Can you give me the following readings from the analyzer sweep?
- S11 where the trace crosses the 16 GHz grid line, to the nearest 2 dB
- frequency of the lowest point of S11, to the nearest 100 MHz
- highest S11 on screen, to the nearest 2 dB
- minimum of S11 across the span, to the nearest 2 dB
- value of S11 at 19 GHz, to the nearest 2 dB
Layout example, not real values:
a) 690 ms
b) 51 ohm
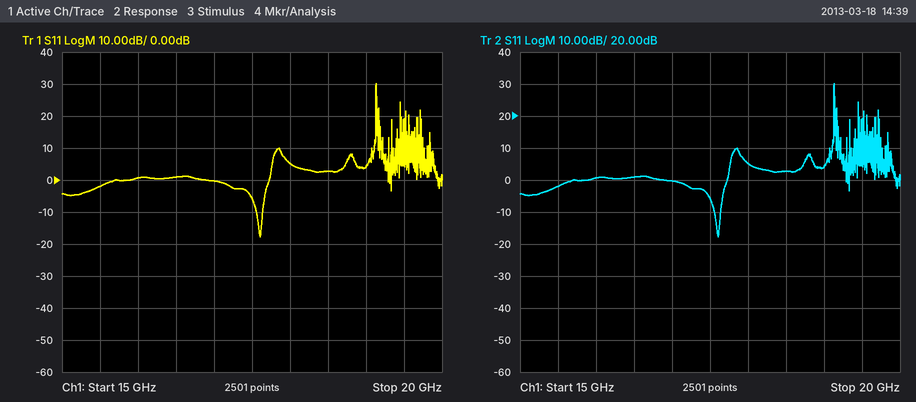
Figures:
a) 0 dB
b) 17.6 GHz
c) 30 dB
d) -18 dB
e) 4 dB
